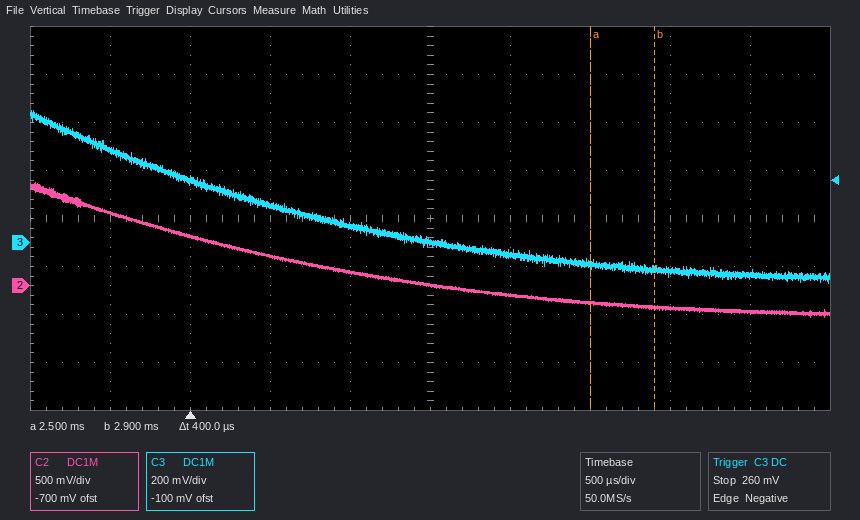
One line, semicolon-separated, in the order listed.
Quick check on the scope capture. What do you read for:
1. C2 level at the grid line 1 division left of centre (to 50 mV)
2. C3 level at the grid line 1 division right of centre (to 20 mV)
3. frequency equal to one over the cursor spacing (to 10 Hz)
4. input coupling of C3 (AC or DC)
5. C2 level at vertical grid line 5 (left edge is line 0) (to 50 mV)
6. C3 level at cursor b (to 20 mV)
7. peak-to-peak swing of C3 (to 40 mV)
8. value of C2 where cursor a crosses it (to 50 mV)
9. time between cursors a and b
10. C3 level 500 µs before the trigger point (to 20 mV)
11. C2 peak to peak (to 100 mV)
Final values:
150 mV; -40 mV; 2.50 kHz; DC; 0 mV; -120 mV; 720 mV; -200 mV; 400 µs; 380 mV; 1.40 V
